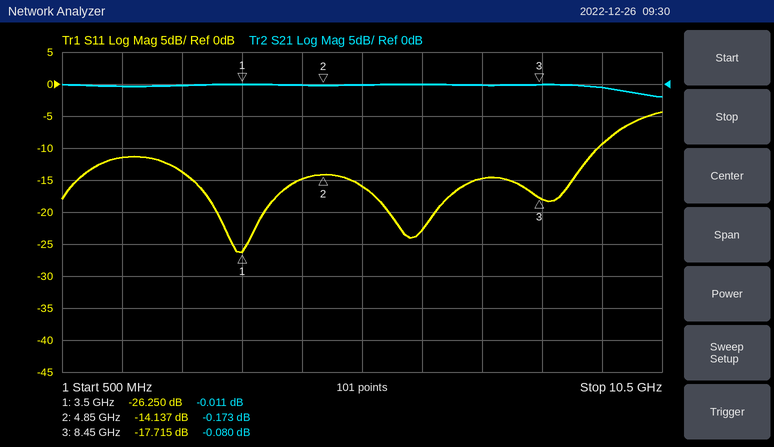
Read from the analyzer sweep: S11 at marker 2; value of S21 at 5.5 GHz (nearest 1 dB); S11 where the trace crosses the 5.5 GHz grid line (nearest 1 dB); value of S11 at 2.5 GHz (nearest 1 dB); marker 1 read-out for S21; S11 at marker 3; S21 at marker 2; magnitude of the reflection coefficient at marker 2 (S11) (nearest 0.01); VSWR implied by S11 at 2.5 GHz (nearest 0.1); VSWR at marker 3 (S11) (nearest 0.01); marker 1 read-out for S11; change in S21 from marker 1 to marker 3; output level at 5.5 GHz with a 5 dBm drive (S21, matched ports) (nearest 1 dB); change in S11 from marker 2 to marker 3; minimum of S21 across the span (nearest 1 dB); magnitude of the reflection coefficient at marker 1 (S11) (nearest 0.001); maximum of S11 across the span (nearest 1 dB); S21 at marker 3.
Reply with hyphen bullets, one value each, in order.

- -14.137 dB
- 0 dB
- -16 dB
- -14 dB
- -0.011 dB
- -17.715 dB
- -0.173 dB
- 0.20
- 1.5
- 1.30
- -26.250 dB
- -0.069 dB
- 5 dBm
- -3.578 dB
- -2 dB
- 0.049
- -4 dB
- -0.080 dB
